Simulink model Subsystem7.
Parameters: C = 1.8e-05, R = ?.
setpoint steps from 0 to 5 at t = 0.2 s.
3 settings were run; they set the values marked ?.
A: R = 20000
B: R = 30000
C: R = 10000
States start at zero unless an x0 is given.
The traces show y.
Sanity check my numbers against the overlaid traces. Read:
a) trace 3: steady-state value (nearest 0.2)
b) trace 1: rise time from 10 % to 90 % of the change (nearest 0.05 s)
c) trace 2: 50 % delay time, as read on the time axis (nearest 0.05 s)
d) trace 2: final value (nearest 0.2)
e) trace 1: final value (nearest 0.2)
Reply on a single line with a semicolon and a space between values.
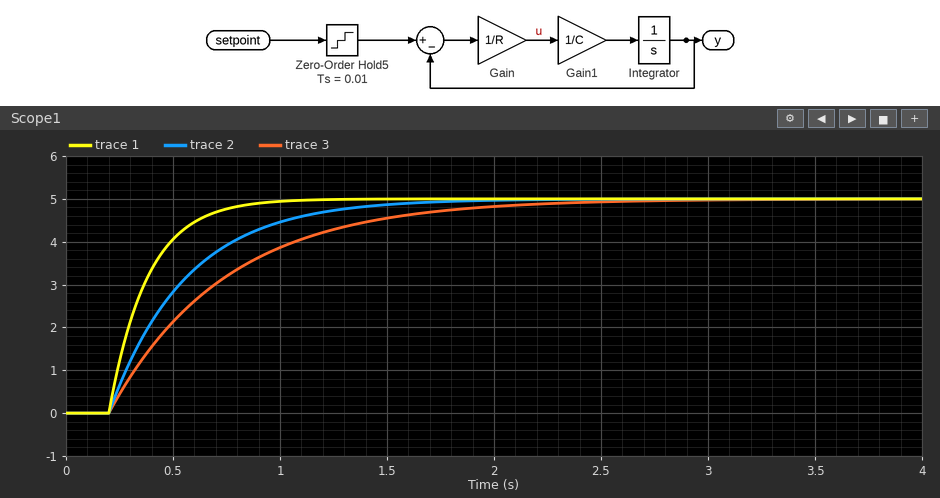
5.0; 0.40 s; 0.45 s; 5.0; 5.0
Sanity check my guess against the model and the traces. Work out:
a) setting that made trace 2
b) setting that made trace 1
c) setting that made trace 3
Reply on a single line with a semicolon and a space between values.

A; C; B
